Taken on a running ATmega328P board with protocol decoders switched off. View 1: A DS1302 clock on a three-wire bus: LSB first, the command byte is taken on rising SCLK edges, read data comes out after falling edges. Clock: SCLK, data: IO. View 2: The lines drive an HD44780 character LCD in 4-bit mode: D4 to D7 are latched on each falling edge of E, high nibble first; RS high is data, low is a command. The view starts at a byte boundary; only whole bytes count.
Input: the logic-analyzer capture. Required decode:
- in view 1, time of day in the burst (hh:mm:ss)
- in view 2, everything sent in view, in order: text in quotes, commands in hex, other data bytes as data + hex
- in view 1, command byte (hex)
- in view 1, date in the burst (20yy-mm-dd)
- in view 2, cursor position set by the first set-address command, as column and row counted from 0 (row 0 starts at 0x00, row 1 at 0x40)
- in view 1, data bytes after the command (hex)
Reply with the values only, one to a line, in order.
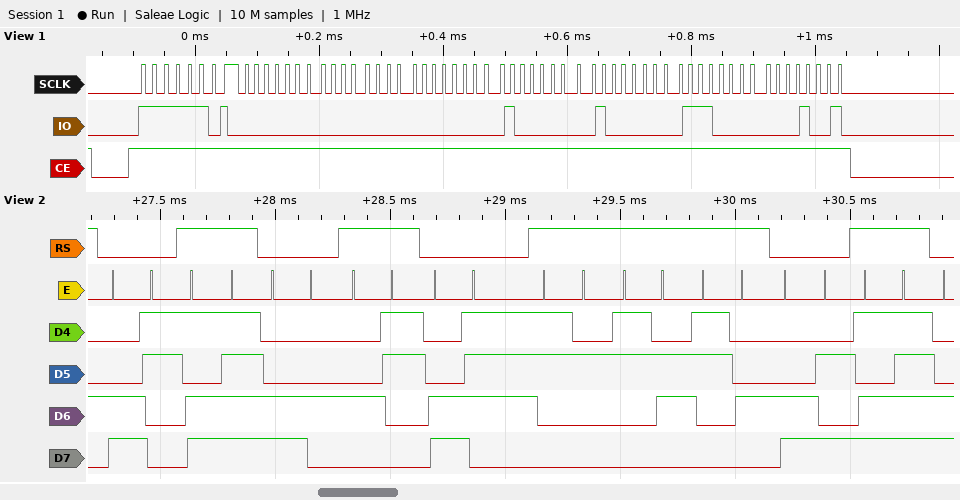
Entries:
00:00:00
0xC3 data DF 0xC4 "C" 0xC7 "264" 0xCA data DF
0xBF
2048-01-01
column 3, row 1
00 00 00 01 01 07 48
